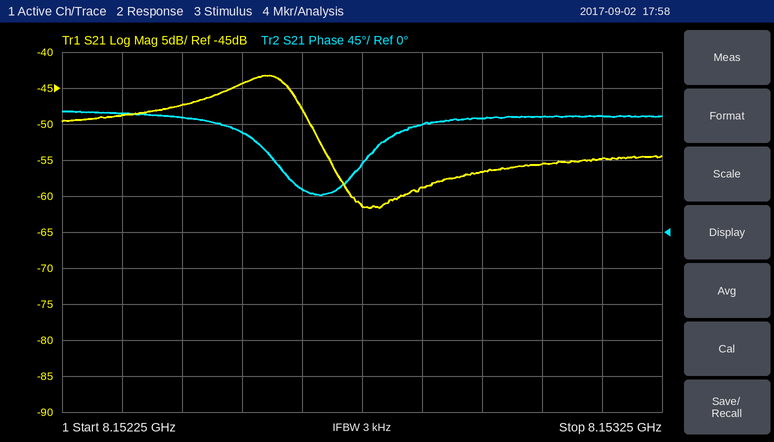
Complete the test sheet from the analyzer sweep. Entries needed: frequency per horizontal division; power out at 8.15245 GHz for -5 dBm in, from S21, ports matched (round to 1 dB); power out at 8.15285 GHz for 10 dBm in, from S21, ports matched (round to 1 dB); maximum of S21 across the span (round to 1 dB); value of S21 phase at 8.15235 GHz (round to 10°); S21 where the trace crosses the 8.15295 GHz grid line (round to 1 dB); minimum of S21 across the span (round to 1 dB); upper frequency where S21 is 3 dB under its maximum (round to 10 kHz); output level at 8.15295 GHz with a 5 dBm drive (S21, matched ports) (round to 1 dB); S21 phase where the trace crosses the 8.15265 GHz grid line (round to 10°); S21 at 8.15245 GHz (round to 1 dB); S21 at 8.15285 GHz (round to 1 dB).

100 kHz
-52 dBm
-49 dBm
-43 dB
150°
-57 dB
-62 dB
8.15264 GHz
-52 dBm
50°
-47 dB
-59 dB
